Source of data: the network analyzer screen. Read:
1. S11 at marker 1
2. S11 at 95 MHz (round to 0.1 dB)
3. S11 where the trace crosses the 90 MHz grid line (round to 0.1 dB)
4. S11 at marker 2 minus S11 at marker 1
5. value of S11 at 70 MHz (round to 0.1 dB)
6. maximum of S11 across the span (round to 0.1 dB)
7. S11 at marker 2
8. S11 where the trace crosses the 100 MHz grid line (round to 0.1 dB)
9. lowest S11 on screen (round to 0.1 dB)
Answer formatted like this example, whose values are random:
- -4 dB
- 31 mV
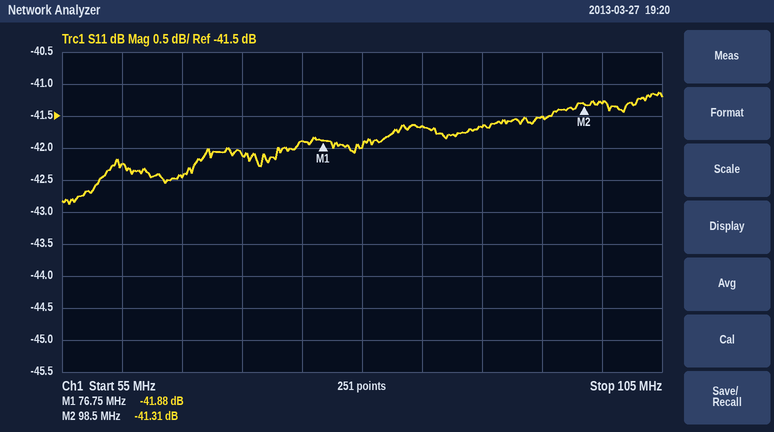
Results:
- -41.88 dB
- -41.5 dB
- -41.7 dB
- 0.57 dB
- -42.1 dB
- -41.1 dB
- -41.31 dB
- -41.3 dB
- -42.9 dB
